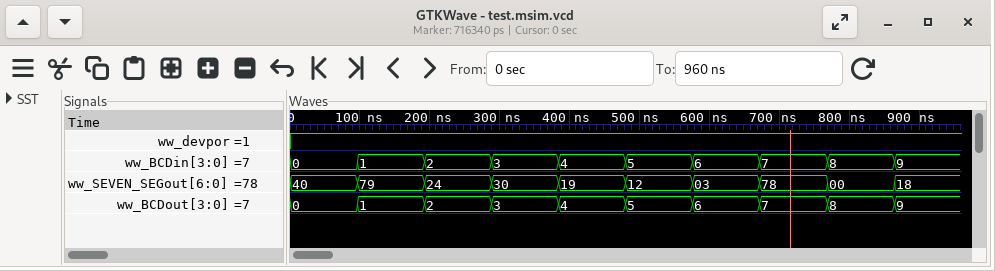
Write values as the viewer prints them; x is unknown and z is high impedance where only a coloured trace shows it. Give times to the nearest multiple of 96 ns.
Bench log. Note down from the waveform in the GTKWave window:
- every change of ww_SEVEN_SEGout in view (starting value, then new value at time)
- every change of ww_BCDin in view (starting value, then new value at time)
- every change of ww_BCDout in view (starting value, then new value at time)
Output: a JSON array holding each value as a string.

["40, 79 at 96 ns, 24 at 192 ns, 30 at 288 ns, 19 at 384 ns, 12 at 480 ns, 03 at 576 ns, 78 at 672 ns, 00 at 768 ns, 18 at 864 ns", "0, 1 at 96 ns, 2 at 192 ns, 3 at 288 ns, 4 at 384 ns, 5 at 480 ns, 6 at 576 ns, 7 at 672 ns, 8 at 768 ns, 9 at 864 ns", "0, 1 at 96 ns, 2 at 192 ns, 3 at 288 ns, 4 at 384 ns, 5 at 480 ns, 6 at 576 ns, 7 at 672 ns, 8 at 768 ns, 9 at 864 ns"]
